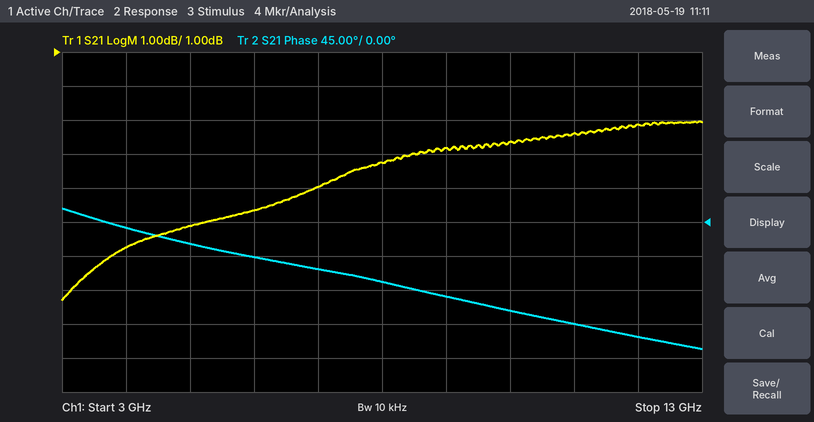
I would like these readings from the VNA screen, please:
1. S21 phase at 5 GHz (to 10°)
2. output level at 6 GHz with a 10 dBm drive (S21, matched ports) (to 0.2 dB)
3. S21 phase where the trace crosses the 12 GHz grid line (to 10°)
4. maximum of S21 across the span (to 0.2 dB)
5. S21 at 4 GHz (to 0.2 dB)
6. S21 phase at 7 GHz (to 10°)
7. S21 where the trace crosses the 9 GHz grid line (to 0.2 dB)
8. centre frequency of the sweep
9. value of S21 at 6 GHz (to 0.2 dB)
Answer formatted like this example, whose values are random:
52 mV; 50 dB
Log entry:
-30°; 6.4 dBm; -150°; -1.0 dB; -4.8 dB; -60°; -1.8 dB; 8 GHz; -3.6 dB
